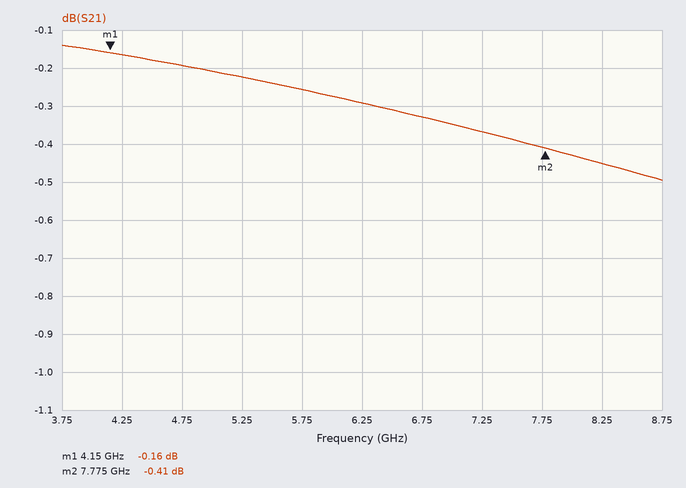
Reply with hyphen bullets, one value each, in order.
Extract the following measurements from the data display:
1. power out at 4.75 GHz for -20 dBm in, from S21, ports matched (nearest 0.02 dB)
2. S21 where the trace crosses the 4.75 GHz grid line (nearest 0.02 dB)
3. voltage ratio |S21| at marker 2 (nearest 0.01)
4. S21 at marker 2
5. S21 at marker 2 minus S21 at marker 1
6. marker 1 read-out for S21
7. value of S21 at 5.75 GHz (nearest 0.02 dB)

- -20.20 dBm
- -0.20 dB
- 0.95
- -0.41 dB
- -0.25 dB
- -0.16 dB
- -0.26 dB
